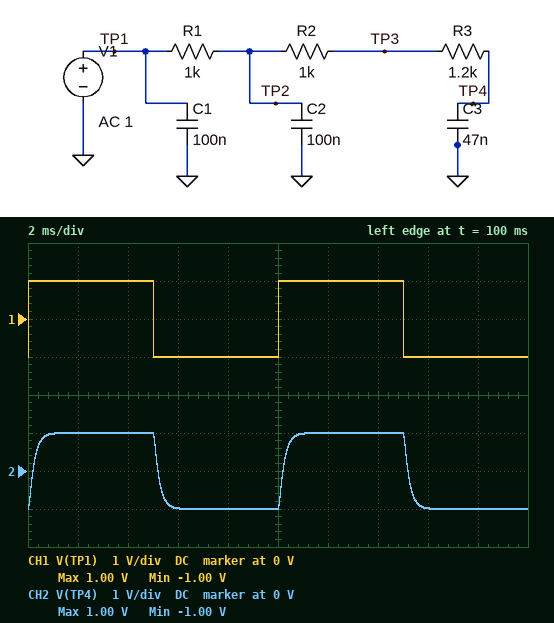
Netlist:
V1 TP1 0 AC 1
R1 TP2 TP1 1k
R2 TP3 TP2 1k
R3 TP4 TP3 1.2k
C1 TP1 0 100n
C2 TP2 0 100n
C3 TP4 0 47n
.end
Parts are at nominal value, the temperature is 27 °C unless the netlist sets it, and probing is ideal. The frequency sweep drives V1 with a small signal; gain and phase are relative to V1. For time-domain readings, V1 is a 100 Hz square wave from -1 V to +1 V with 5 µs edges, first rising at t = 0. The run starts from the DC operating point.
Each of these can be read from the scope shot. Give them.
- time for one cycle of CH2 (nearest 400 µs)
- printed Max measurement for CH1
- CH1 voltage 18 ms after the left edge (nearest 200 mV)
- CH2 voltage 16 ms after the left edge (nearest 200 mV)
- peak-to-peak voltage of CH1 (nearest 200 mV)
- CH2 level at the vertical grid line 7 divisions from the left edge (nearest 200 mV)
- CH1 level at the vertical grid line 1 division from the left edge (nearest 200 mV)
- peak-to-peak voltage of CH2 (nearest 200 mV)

10.0 ms
1.00 V
-1.0 V
-1.0 V
2.0 V
1.0 V
1.0 V
2.0 V
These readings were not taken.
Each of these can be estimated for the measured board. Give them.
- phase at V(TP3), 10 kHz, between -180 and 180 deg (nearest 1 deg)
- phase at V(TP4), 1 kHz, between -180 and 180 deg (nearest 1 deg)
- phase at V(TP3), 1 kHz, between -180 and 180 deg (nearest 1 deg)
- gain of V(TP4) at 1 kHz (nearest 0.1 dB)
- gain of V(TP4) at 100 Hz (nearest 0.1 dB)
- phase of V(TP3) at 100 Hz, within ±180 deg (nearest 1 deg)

-84 deg
-69 deg
-50 deg
-4.5 dB
-0.1 dB
-7 deg
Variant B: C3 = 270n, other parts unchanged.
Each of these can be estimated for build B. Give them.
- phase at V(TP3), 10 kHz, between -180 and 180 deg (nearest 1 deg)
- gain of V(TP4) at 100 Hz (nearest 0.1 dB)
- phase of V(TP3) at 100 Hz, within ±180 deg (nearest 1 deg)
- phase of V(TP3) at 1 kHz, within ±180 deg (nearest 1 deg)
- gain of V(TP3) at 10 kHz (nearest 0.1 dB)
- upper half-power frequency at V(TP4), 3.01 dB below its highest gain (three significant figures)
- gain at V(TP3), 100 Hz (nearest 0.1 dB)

-78 deg
-1.2 dB
-20 deg
-39 deg
-21.5 dB
176 Hz
-1.0 dB
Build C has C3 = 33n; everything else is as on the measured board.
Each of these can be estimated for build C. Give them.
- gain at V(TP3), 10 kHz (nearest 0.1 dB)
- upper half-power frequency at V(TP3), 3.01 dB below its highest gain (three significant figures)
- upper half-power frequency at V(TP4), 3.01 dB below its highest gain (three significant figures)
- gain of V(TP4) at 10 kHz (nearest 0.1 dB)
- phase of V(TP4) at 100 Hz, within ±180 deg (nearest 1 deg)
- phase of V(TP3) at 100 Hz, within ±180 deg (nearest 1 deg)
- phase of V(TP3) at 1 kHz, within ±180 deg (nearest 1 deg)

-21.1 dB
976 Hz
926 Hz
-29.7 dB
-7 deg
-6 deg
-47 deg
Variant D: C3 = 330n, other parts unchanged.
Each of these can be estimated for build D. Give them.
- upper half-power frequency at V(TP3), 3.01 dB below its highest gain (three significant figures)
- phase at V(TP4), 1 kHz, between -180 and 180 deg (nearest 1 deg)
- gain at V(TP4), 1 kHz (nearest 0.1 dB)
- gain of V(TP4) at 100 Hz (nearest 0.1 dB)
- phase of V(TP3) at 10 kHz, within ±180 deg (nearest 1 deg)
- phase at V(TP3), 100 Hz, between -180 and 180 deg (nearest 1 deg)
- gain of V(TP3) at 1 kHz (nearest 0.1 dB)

169 Hz
-104 deg
-17.5 dB
-1.7 dB
-78 deg
-23 deg
-8.9 dB
